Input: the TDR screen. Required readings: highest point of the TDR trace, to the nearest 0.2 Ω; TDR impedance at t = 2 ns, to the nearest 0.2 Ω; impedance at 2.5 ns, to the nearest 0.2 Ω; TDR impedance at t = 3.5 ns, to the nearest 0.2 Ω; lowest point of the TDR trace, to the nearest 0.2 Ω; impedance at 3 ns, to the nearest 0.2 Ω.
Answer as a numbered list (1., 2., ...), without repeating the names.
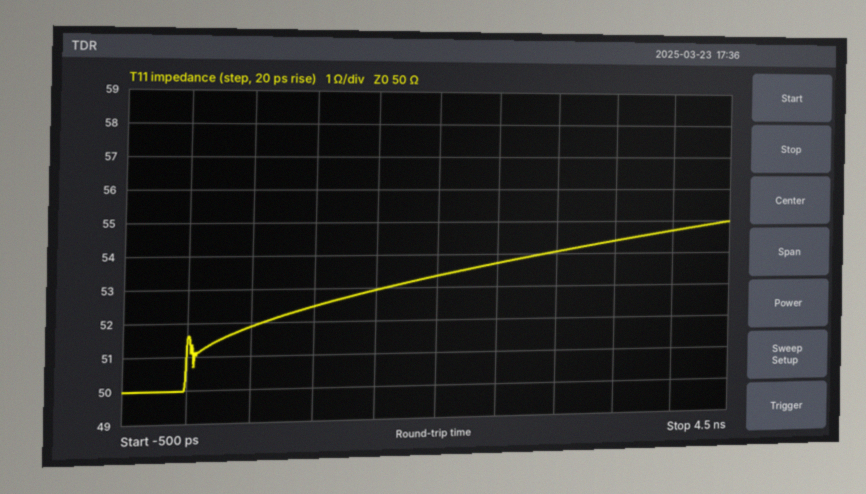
1. 55.0 Ω
2. 53.4 Ω
3. 53.8 Ω
4. 54.4 Ω
5. 50.0 Ω
6. 54.0 Ω
